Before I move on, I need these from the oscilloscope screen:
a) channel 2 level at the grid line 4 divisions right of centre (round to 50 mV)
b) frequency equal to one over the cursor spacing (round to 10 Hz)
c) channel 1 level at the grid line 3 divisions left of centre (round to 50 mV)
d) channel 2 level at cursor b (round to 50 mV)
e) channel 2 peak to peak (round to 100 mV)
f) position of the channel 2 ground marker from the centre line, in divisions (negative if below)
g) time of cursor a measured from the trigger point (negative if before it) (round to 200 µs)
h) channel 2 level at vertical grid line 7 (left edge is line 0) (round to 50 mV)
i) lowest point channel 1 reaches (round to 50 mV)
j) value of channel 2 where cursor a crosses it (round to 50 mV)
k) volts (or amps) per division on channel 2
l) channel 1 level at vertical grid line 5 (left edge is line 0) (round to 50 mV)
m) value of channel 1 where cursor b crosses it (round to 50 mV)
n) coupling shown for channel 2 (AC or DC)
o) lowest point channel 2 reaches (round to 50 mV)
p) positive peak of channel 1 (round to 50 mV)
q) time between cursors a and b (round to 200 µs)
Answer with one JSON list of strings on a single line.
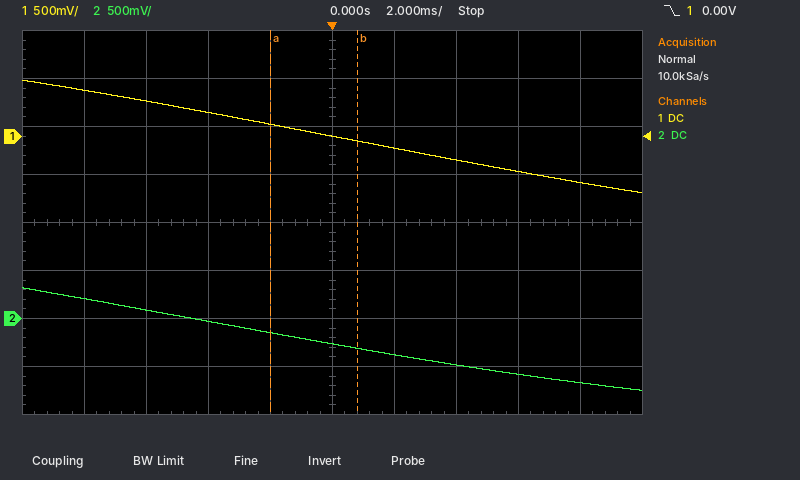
["-650 mV", "360 Hz", "350 mV", "-300 mV", "1.10 V", "-2.0 div", "-2.0 ms", "-500 mV", "-600 mV", "-150 mV", "500 mV", "0 mV", "-50 mV", "DC", "-750 mV", "600 mV", "2.8 ms"]
